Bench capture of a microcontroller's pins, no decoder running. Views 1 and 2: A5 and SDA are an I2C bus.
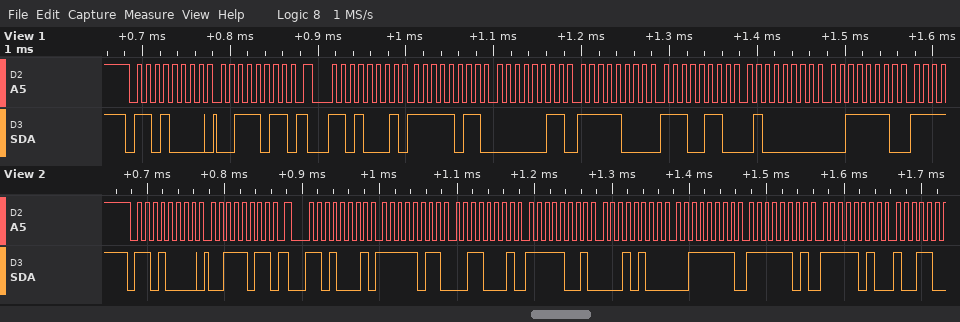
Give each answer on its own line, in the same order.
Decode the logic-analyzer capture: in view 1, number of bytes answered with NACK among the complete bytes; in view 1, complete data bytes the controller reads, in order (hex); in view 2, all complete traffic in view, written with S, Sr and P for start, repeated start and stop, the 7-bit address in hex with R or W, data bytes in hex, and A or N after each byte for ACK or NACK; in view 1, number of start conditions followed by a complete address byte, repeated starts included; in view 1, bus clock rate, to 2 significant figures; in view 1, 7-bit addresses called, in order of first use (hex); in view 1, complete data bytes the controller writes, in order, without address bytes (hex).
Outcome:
0
FB 03 F8 E6 40 3E
S 68W A 3B A Sr 68R A FB A 31 A F9 A 14 A 3F A FD A FA A
2
100 kHz
0x68
3B
